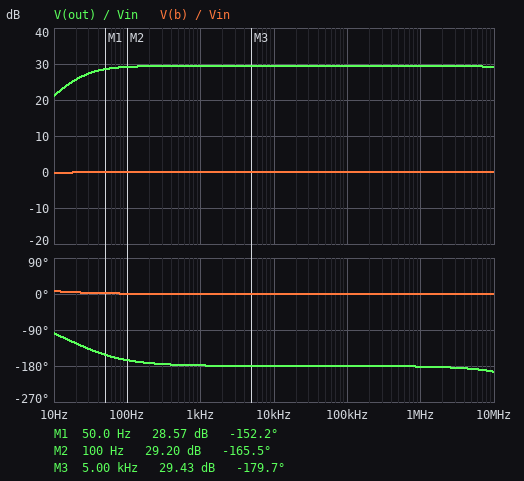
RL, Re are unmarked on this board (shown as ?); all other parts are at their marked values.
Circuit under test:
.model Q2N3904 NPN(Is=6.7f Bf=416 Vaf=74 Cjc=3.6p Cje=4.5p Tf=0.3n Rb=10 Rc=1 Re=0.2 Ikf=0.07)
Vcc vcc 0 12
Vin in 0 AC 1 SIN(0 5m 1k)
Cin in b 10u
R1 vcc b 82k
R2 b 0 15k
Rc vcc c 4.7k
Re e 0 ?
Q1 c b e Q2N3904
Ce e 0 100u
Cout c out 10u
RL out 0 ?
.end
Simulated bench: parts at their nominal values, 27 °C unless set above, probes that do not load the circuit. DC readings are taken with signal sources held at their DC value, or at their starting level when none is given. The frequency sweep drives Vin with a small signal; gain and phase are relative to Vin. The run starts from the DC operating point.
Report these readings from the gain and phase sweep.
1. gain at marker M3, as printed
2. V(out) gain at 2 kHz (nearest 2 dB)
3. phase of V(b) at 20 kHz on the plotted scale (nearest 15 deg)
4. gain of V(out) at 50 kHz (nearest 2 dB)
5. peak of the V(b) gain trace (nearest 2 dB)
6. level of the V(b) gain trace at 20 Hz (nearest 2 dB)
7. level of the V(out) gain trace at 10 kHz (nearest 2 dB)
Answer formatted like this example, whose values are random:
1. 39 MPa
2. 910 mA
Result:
1. 29.43 dB
2. 30 dB
3. 0 deg
4. 30 dB
5. 0 dB
6. 0 dB
7. 30 dB
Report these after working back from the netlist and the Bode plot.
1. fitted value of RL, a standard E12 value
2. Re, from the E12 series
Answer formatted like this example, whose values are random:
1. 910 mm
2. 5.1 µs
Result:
1. 3.9 kΩ
2. 3.3 kΩ
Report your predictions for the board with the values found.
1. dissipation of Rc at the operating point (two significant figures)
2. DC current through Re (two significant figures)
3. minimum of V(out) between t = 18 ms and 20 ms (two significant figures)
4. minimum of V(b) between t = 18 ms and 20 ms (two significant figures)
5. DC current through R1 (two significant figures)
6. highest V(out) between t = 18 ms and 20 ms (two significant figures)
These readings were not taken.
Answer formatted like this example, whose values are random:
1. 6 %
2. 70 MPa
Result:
1. 630 µW
2. 370 µA
3. -150 mV
4. 1.8 V
5. 120 µA
6. 140 mV
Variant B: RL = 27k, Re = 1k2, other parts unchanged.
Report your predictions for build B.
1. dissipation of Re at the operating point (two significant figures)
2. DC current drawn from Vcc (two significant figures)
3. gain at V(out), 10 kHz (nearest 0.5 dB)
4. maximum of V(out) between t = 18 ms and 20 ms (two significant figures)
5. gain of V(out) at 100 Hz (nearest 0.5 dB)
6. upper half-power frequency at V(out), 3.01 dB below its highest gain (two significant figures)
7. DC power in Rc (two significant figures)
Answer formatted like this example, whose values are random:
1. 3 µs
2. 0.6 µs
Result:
1. 1.1 mW
2. 1.1 mA
3. 43.0 dB
4. 670 mV
5. 41.5 dB
6. 17 MHz
7. 4.4 mW
